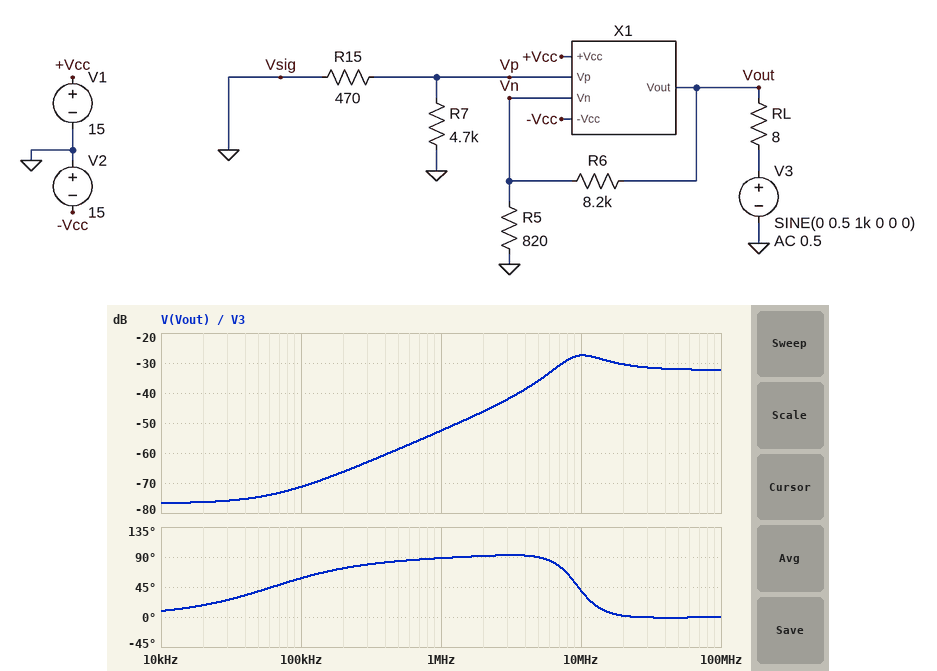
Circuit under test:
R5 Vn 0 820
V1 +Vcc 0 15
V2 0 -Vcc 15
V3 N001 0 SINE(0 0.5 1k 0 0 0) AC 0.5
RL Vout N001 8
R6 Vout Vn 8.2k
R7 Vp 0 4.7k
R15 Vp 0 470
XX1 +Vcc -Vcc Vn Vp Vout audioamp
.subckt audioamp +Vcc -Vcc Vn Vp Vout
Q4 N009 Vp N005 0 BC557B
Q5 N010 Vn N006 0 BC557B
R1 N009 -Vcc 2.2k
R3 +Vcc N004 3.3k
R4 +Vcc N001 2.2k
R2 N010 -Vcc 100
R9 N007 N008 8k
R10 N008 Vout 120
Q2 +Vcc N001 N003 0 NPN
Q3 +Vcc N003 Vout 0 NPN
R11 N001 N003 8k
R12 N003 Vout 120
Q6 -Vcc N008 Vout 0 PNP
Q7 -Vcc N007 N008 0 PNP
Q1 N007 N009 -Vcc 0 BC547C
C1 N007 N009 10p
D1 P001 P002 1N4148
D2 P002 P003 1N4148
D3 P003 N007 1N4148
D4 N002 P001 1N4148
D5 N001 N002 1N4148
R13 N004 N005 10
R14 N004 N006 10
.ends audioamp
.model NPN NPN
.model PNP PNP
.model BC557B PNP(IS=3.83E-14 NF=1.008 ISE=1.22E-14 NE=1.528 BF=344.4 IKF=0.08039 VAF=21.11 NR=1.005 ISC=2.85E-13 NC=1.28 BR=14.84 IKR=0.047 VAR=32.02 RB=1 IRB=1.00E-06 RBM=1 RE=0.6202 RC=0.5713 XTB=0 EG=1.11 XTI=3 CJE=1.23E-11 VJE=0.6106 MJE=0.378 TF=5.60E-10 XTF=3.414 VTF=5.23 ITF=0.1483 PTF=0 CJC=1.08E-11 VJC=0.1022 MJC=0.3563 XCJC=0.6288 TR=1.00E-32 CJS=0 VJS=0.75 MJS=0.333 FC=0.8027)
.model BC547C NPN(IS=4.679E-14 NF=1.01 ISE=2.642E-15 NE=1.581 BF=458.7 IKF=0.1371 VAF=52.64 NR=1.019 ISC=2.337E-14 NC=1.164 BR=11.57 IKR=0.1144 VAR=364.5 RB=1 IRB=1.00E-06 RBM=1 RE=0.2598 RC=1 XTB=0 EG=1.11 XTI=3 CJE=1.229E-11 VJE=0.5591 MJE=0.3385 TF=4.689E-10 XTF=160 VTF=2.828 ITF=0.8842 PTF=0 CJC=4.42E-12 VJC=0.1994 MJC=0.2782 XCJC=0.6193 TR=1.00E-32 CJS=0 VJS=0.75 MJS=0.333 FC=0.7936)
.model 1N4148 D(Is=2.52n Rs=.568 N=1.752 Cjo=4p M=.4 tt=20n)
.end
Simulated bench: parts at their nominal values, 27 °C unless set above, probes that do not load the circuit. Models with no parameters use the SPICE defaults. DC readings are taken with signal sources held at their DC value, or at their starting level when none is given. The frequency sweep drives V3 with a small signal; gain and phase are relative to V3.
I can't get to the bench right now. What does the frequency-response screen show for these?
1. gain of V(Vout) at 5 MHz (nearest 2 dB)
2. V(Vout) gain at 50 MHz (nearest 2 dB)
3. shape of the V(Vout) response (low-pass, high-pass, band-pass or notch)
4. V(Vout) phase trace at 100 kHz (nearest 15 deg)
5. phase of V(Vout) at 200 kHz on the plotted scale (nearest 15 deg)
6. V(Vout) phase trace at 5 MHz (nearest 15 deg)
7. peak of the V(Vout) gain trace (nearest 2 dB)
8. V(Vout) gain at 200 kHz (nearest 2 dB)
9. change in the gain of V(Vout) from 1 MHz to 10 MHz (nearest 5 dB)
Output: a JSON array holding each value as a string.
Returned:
["-36 dB", "-32 dB", "high-pass", "60 deg", "75 deg", "90 deg", "-28 dB", "-66 dB", "25 dB"]
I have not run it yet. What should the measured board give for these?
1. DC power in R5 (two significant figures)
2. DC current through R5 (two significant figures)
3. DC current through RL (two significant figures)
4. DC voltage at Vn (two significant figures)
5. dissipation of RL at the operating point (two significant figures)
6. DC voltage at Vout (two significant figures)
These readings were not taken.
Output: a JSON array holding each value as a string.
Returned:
["14 µW", "130 µA", "150 mA", "-110 mV", "190 mW", "-1.2 V"]
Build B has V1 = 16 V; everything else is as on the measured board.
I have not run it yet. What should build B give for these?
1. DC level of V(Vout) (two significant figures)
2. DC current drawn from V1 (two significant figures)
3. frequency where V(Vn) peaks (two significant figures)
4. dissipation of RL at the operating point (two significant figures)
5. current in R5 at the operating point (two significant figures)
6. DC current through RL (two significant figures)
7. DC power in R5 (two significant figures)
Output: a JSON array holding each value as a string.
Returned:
["-1.3 V", "24 mA", "10 MHz", "210 mW", "140 µA", "160 mA", "15 µW"]
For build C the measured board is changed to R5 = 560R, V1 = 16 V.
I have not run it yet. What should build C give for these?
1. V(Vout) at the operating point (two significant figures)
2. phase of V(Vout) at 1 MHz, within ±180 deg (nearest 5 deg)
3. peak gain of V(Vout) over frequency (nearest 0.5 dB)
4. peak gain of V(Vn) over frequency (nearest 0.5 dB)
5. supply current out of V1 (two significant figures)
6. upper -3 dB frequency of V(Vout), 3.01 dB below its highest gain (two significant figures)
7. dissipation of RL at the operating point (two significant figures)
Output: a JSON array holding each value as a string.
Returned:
["-1.8 V", "85 deg", "-31.5 dB", "-56.5 dB", "24 mA", "35 MHz", "410 mW"]
